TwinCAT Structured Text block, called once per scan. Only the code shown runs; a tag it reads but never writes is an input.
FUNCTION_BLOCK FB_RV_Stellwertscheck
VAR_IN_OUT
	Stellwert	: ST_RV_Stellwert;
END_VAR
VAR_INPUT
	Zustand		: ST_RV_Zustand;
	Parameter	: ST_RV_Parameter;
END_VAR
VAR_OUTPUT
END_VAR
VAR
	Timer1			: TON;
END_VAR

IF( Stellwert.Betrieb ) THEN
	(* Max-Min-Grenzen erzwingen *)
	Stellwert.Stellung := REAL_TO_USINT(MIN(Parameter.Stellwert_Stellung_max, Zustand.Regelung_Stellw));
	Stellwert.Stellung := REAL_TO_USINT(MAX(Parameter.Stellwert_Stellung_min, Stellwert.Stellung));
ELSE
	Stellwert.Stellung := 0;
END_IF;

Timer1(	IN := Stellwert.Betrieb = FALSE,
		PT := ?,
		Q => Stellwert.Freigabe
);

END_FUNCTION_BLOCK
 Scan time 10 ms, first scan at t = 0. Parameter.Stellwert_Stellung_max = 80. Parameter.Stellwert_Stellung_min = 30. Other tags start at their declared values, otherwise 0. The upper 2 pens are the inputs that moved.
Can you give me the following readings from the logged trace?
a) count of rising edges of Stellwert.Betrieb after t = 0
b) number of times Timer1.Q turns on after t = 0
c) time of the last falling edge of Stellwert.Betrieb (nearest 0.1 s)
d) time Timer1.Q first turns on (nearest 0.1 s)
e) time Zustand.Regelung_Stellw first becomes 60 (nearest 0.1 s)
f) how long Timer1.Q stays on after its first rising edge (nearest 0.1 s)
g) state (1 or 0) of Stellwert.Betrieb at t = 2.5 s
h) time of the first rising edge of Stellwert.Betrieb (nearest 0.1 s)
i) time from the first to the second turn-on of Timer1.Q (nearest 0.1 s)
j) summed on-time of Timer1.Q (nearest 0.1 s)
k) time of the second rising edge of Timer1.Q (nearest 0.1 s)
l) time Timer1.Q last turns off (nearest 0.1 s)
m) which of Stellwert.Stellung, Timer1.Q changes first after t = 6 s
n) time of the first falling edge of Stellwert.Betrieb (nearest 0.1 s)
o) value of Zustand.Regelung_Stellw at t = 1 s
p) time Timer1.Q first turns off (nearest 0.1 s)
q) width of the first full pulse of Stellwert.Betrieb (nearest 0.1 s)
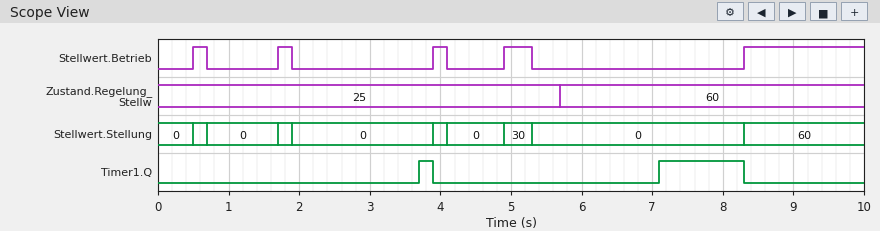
5
2
5.3 s
3.7 s
5.7 s
0.2 s
0
0.5 s
3.4 s
1.4 s
7.1 s
8.3 s
Timer1.Q
0.7 s
25
3.9 s
0.2 s
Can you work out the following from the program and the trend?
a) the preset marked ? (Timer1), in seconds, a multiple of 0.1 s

1.8 s
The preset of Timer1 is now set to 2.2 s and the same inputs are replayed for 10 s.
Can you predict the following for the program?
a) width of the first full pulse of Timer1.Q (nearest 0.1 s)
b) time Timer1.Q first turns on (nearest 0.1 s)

0.8 s
7.5 s
